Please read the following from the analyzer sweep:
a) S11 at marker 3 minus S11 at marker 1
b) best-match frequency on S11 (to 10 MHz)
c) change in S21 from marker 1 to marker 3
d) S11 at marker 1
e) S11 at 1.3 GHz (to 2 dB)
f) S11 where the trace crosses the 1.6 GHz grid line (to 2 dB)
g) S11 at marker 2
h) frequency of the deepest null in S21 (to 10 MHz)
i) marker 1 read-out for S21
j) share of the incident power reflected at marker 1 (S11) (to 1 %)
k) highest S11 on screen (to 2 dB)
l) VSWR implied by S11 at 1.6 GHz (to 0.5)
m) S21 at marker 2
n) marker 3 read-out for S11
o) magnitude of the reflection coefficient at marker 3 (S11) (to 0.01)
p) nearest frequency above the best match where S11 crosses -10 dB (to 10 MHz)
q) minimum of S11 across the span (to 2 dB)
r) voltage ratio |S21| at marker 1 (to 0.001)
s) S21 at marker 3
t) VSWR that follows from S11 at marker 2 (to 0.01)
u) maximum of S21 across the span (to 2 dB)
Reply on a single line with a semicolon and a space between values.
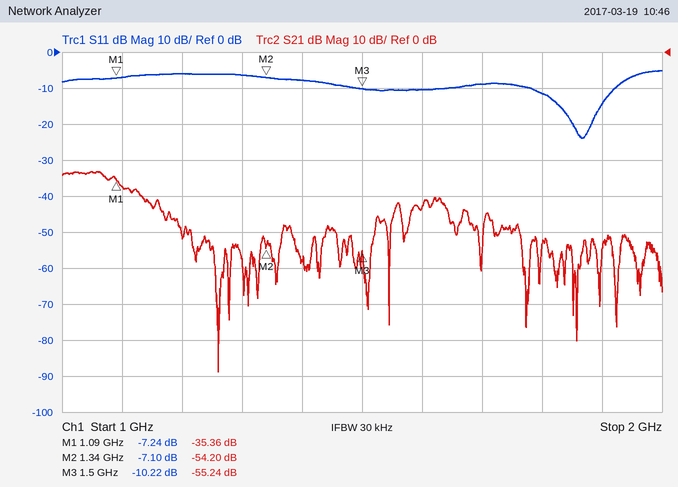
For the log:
-2.98 dB; 1.87 GHz; -19.88 dB; -7.24 dB; -6 dB; -10 dB; -7.10 dB; 1.26 GHz; -35.36 dB; 19 %; -6 dB; 2.0; -54.20 dB; -10.22 dB; 0.31; 1.92 GHz; -24 dB; 0.017; -55.24 dB; 2.58; -34 dB
